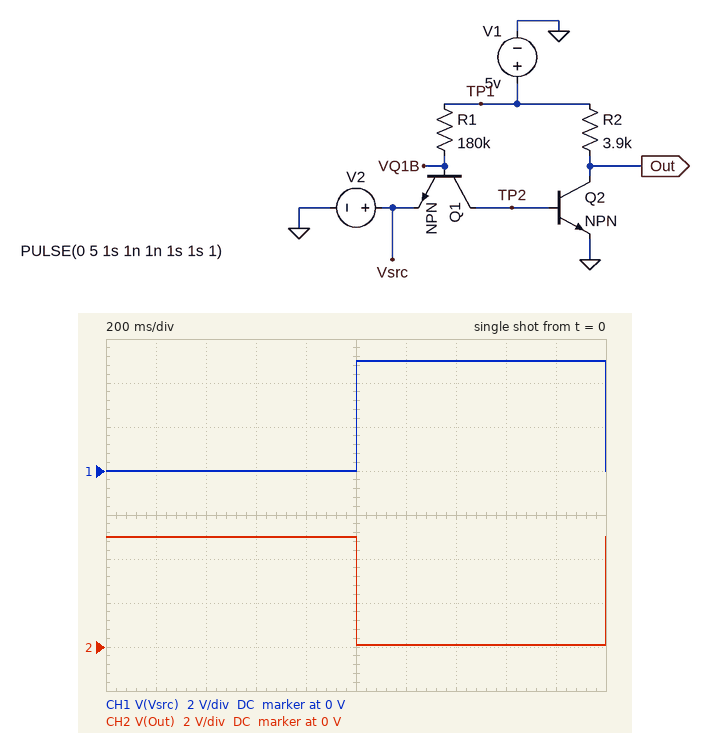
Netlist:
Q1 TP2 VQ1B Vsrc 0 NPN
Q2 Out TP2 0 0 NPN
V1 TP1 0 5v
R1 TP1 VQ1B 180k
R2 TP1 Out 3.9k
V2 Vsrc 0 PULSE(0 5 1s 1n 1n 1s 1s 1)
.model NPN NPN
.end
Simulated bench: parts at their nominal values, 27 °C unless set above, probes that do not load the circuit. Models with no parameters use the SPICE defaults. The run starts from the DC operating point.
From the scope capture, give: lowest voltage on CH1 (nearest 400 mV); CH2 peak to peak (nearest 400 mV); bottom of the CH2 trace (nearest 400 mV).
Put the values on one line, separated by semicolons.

0 V; 4.8 V; 0 V
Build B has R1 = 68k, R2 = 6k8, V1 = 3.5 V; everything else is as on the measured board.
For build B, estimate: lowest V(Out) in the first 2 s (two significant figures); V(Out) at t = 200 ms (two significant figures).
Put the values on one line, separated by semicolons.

63 mV; 3.5 V
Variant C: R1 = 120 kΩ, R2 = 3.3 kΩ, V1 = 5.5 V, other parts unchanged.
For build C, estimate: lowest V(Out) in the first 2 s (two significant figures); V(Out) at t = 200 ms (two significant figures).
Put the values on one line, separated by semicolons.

92 mV; 5.5 V
